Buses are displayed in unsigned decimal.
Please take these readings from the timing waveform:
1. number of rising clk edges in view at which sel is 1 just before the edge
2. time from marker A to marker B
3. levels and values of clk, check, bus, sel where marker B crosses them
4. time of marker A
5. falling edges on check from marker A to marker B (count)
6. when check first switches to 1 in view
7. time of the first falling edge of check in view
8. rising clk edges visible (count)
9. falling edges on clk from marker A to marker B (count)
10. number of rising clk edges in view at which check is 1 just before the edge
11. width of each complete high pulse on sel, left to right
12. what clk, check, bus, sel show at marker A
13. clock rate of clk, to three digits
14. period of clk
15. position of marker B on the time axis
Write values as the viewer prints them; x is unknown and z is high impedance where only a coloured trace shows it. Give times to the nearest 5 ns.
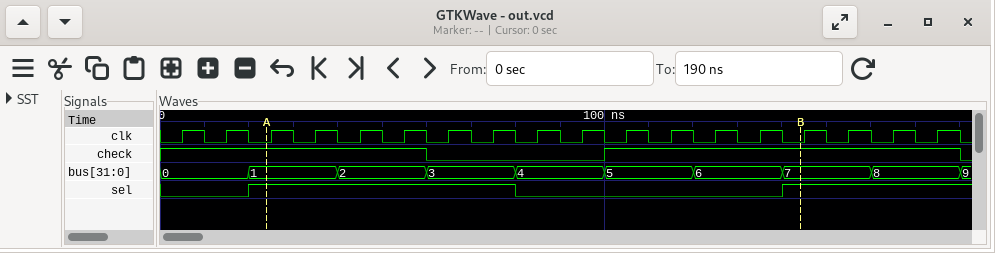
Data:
10
120 ns
clk=0, check=1, bus=7, sel=1
25 ns
1
100 ns
60 ns
18
12
14
60 ns
clk=0, check=1, bus=1, sel=1
100 MHz
10 ns
145 ns
